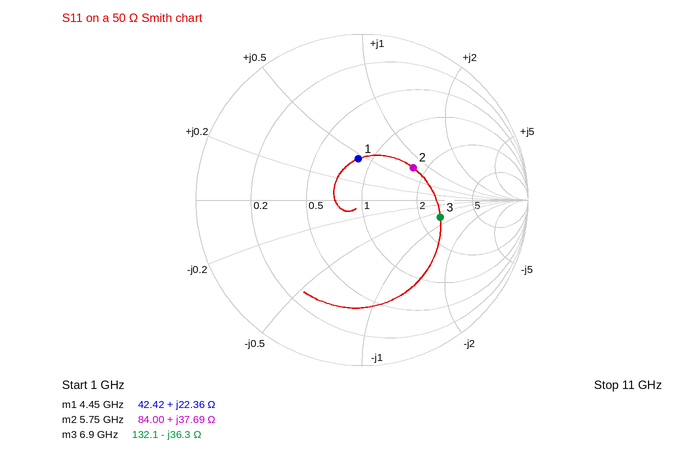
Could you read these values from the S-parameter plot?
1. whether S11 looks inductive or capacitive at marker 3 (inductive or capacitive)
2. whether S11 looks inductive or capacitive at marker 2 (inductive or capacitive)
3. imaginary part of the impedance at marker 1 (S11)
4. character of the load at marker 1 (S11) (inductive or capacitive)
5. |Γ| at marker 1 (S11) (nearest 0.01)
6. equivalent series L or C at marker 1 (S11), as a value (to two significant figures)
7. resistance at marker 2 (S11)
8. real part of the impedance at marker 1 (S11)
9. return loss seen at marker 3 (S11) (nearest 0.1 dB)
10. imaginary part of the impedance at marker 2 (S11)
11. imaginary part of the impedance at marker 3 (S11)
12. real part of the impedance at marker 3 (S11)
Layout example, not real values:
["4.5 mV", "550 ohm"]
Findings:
["capacitive", "inductive", "+22.36 Ω", "inductive", "0.25", "800 pH", "84.00 Ω", "42.42 Ω", "6.3 dB", "+37.69 Ω", "-36.3 Ω", "132.1 Ω"]
